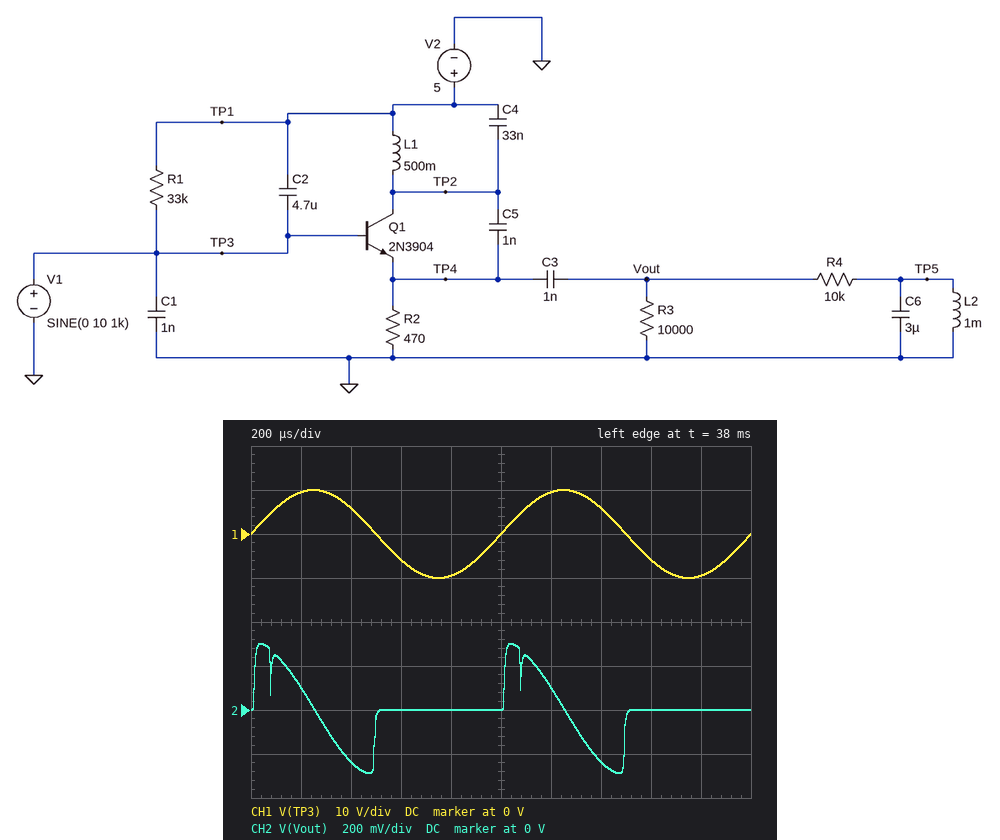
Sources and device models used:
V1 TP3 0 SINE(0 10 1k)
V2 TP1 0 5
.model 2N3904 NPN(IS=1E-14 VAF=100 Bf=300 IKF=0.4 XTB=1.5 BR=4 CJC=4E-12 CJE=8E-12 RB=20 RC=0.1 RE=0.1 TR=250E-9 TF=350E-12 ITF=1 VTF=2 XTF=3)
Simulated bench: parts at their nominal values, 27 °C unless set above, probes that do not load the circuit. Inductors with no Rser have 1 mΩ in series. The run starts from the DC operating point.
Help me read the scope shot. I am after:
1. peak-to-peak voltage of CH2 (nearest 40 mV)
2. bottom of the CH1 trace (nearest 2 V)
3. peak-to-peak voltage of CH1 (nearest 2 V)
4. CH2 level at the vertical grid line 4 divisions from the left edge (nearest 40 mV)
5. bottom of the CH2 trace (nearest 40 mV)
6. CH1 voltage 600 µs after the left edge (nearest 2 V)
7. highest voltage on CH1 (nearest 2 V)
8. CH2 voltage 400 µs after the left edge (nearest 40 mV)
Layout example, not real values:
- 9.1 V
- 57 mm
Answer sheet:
- 600 mV
- -10 V
- 20 V
- 0 V
- -280 mV
- -6 V
- 10 V
- -240 mV
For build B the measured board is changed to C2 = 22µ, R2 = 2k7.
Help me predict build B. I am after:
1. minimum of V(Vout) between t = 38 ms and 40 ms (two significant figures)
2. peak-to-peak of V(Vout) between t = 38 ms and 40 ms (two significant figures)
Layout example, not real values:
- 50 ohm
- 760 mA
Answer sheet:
- -300 mV
- 600 mV
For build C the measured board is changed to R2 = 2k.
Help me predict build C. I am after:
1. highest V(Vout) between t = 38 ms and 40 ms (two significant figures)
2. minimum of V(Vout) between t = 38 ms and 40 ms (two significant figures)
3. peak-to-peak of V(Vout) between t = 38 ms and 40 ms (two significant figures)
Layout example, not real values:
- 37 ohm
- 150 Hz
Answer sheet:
- 300 mV
- -300 mV
- 600 mV
